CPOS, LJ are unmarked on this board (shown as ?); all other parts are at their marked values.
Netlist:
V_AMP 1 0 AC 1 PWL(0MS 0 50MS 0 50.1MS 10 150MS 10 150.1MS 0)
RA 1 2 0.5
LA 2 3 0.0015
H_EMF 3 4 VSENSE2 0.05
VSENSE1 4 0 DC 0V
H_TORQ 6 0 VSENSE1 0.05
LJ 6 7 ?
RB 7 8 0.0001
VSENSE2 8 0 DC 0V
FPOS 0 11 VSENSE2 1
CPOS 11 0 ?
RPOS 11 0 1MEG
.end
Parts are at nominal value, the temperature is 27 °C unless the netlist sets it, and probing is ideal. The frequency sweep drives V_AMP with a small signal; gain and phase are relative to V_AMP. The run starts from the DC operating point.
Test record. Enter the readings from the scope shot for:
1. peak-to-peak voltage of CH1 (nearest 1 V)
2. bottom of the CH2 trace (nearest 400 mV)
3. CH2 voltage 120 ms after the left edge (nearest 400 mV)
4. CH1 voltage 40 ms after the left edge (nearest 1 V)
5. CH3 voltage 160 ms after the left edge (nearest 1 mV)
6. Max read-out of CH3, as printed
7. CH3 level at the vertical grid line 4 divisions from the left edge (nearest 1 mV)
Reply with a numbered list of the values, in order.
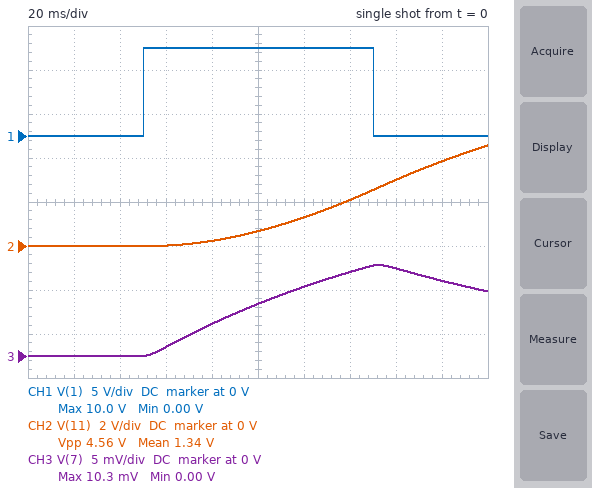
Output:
1. 10 V
2. 0 V
3. 1.2 V
4. 0 V
5. 10 mV
6. 10.3 mV
7. 4 mV
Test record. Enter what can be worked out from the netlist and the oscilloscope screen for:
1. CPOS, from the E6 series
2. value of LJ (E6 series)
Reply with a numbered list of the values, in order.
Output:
1. 2.2 F
2. 680 µH
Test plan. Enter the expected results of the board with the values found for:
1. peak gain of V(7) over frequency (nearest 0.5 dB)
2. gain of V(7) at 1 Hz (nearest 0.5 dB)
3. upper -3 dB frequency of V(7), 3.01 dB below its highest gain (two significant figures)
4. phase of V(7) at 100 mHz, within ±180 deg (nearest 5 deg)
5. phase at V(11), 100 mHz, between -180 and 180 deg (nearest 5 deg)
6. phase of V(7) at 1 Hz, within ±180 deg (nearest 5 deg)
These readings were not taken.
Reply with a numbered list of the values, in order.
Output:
1. -54.0 dB
2. -56.5 dB
3. 1.2 Hz
4. -5 deg
5. -95 deg
6. -40 deg
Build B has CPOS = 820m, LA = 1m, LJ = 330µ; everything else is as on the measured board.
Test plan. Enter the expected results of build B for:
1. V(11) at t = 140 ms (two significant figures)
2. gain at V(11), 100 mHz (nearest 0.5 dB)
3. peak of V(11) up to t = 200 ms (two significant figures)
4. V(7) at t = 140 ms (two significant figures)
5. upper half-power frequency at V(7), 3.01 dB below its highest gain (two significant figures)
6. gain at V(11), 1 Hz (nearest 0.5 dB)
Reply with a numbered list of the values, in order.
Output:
1. 9.7 V
2. 31.5 dB
3. 18 V
4. 15 mV
5. 2.5 Hz
6. 11.0 dB
